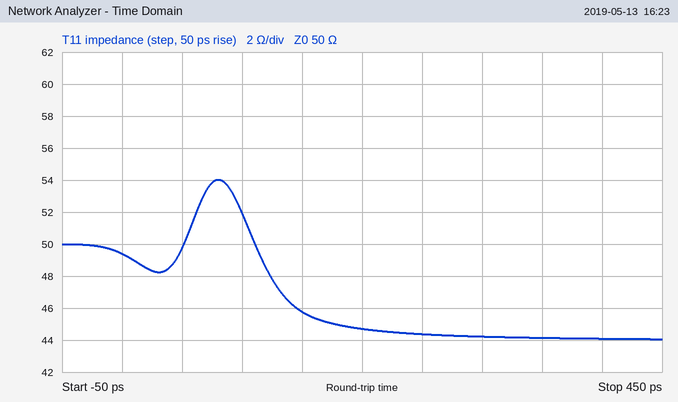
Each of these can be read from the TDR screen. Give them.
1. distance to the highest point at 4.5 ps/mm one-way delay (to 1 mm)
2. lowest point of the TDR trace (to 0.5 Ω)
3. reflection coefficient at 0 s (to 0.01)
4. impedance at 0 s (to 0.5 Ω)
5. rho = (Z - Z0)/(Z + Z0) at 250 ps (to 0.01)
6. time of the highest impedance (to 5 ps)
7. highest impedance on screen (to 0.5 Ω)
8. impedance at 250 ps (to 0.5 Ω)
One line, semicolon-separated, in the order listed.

9 mm; 44.0 Ω; -0.01; 49.5 Ω; -0.06; 80 ps; 54.0 Ω; 44.5 Ω
